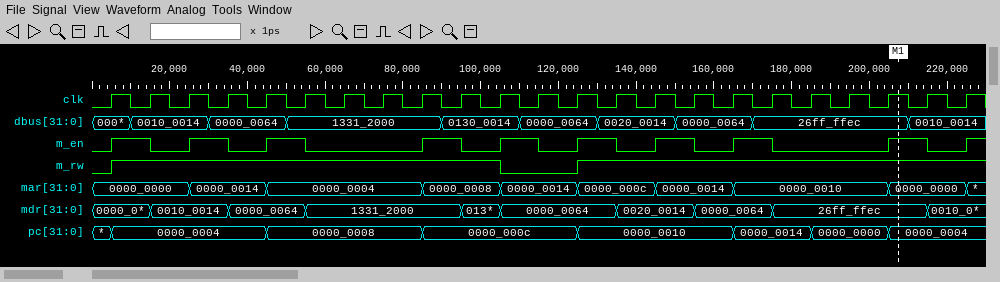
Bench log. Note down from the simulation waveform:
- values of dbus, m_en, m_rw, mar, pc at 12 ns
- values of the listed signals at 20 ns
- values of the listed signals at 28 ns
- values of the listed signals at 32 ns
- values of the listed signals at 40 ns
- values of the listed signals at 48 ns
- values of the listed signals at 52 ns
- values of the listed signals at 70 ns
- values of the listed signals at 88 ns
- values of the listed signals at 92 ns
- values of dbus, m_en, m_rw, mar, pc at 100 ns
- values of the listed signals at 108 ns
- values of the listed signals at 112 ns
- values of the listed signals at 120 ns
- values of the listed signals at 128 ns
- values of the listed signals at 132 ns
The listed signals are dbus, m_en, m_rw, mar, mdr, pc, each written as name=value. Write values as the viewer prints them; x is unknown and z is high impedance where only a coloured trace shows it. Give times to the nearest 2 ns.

dbus=0010_0014, m_en=1, m_rw=1, mar=0000_0000, pc=0000_0004
dbus=0010_0014, m_en=0, m_rw=1, mar=0000_0000, mdr=0010_0014, pc=0000_0004
dbus=0010_0014, m_en=1, m_rw=1, mar=0000_0014, mdr=0010_0014, pc=0000_0004
dbus=0000_0064, m_en=1, m_rw=1, mar=0000_0014, mdr=0010_0014, pc=0000_0004
dbus=0000_0064, m_en=0, m_rw=1, mar=0000_0014, mdr=0000_0064, pc=0000_0004
dbus=0000_0064, m_en=1, m_rw=1, mar=0000_0004, mdr=0000_0064, pc=0000_0008
dbus=1331_2000, m_en=1, m_rw=1, mar=0000_0004, mdr=0000_0064, pc=0000_0008
dbus=1331_2000, m_en=0, m_rw=1, mar=0000_0004, mdr=1331_2000, pc=0000_0008
dbus=1331_2000, m_en=1, m_rw=1, mar=0000_0008, mdr=1331_2000, pc=0000_000c
dbus=0130_0014, m_en=1, m_rw=1, mar=0000_0008, mdr=1331_2000, pc=0000_000c
dbus=0130_0014, m_en=0, m_rw=1, mar=0000_0008, pc=0000_000c
dbus=0130_0014, m_en=1, m_rw=0, mar=0000_0014, mdr=0000_0064, pc=0000_000c
dbus=0000_0064, m_en=1, m_rw=0, mar=0000_0014, mdr=0000_0064, pc=0000_000c
dbus=0000_0064, m_en=0, m_rw=0, mar=0000_0014, mdr=0000_0064, pc=0000_000c
dbus=0000_0064, m_en=1, m_rw=1, mar=0000_000c, mdr=0000_0064, pc=0000_0010
dbus=0020_0014, m_en=1, m_rw=1, mar=0000_000c, mdr=0000_0064, pc=0000_0010
